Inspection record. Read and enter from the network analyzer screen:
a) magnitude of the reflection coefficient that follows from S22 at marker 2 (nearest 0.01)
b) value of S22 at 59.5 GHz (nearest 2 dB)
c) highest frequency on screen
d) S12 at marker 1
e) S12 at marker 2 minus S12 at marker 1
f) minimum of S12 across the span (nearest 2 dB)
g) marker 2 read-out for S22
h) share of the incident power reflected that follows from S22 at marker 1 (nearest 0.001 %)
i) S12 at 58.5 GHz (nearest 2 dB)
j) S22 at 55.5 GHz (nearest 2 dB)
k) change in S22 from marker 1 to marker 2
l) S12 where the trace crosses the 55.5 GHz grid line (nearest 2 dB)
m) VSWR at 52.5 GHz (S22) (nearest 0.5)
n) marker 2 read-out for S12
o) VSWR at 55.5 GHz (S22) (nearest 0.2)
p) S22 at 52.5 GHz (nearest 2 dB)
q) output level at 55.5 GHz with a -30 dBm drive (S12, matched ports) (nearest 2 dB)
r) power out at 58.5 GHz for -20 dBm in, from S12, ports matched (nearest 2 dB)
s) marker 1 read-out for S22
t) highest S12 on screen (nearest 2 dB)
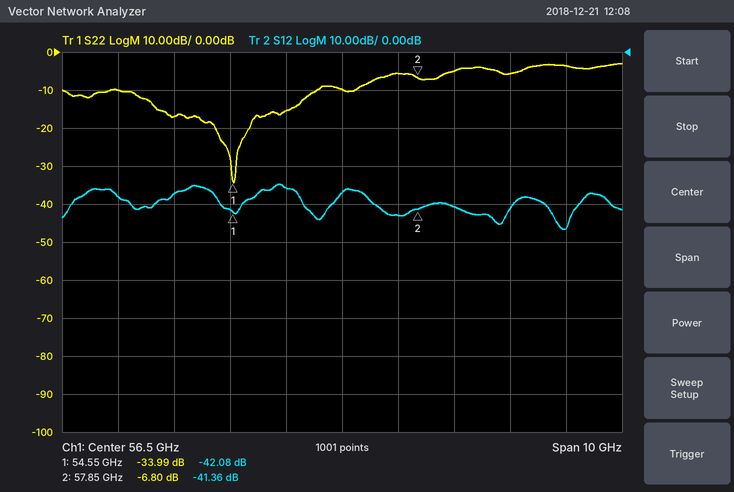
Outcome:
0.46
-6 dB
61.5 GHz
-42.08 dB
0.72 dB
-46 dB
-6.80 dB
0.040 %
-40 dB
-16 dB
27.19 dB
-36 dB
2.0
-41.36 dB
1.4
-10 dB
-66 dBm
-60 dBm
-33.99 dB
-34 dB
